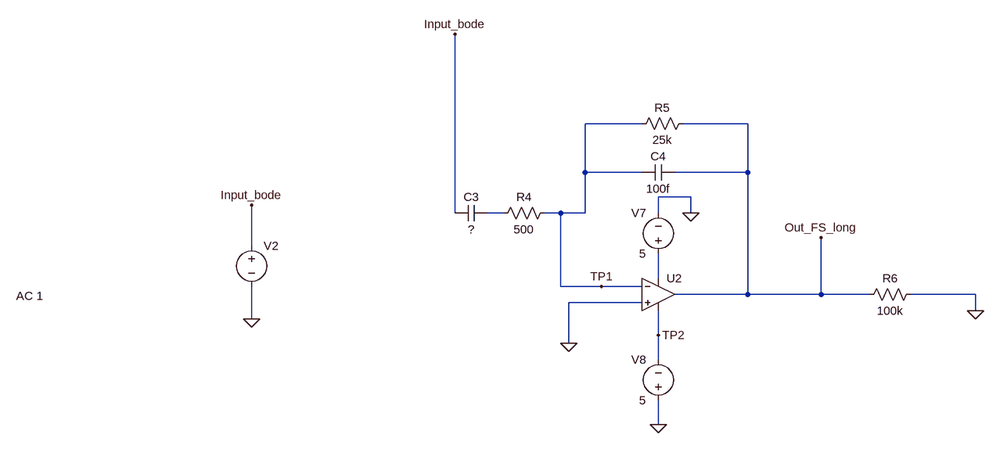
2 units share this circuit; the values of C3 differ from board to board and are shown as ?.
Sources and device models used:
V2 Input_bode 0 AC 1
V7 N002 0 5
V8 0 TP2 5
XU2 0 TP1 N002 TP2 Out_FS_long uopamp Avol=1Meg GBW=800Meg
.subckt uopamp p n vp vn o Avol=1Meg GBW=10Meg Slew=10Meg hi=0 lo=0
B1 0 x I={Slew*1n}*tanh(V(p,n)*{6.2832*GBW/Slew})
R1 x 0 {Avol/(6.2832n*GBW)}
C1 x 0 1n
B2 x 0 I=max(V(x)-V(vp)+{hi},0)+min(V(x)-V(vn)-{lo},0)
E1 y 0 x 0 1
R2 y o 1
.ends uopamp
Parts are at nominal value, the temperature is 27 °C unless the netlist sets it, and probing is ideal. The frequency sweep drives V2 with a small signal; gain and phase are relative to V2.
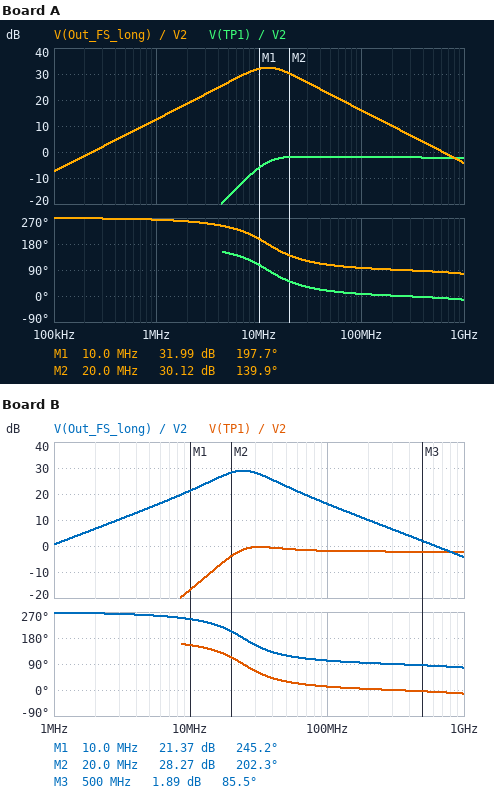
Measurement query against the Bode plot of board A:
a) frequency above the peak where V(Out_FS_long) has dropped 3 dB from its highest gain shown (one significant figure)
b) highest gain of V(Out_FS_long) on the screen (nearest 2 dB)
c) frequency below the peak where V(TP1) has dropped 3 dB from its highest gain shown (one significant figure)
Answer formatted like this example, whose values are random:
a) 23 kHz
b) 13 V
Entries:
a) 20 MHz
b) 32 dB
c) 10 MHz
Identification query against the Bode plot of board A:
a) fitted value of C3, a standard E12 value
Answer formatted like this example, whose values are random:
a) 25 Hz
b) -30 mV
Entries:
a) 27 pF
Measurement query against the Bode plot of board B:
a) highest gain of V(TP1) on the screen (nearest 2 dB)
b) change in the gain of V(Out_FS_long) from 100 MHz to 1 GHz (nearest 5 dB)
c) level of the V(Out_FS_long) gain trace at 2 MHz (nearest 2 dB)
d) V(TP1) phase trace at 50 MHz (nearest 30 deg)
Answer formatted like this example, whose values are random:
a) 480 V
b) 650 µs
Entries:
a) 0 dB
b) -20 dB
c) 6 dB
d) 30 deg
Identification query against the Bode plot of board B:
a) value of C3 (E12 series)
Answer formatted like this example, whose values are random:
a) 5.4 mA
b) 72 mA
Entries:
a) 6.8 pF
